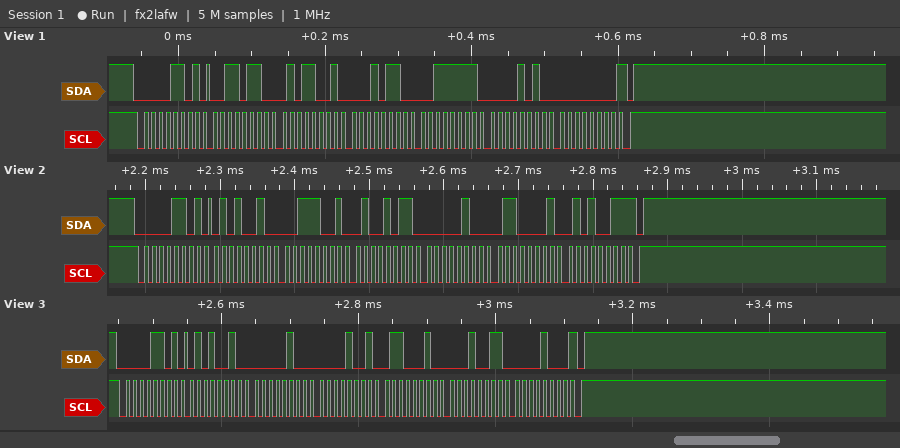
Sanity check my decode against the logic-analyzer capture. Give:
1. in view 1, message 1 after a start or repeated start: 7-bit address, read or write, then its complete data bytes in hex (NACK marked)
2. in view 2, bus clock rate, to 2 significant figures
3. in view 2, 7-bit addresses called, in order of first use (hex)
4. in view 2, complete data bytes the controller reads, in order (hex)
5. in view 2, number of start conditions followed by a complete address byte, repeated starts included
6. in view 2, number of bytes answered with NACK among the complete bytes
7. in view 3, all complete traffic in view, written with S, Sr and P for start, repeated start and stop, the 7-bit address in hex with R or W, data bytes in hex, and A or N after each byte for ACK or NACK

0x06 read: 36 59 16 3F 0A 00 NACK
100 kHz
0x06
52 39 4B 04 61 53
1
1
S 06R A 52 A 04 A 09 A 62 A 13 A 08 N P
